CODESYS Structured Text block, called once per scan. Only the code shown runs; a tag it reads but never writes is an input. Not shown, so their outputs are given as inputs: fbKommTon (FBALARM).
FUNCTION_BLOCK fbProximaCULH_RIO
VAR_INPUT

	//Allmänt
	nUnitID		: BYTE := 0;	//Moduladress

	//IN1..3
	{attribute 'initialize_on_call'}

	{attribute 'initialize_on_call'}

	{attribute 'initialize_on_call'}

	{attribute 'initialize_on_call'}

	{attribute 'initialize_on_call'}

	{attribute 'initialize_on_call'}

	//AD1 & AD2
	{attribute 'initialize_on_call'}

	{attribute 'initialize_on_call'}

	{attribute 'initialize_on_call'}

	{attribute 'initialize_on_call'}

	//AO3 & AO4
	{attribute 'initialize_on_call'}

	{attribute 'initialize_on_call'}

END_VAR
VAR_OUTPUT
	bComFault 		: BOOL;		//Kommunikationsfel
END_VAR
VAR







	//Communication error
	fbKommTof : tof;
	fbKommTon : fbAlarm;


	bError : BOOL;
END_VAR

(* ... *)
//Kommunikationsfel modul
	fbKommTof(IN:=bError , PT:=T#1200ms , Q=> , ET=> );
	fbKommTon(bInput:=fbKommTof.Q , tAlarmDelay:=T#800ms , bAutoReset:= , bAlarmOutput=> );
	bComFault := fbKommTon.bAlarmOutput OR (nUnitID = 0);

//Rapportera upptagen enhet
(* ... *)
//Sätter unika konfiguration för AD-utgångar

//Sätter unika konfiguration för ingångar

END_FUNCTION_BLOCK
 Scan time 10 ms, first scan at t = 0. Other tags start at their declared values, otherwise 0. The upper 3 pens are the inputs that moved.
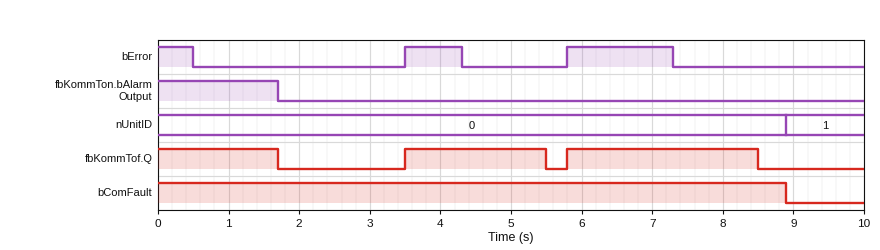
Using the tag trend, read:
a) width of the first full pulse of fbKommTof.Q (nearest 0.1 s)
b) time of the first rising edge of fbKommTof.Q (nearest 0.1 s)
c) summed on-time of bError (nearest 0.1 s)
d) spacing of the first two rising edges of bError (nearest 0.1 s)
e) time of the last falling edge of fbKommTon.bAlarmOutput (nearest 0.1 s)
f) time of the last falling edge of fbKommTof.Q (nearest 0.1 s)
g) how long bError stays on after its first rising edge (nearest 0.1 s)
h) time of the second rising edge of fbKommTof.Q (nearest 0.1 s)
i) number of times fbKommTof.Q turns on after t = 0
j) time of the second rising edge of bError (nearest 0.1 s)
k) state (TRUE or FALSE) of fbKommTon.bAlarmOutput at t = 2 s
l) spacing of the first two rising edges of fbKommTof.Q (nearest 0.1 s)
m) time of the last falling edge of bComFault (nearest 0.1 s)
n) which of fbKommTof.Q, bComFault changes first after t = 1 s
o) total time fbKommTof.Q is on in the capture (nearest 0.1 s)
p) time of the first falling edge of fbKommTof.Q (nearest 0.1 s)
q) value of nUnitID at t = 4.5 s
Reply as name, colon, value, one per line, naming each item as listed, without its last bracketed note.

width of the first full pulse of fbKommTof.Q: 2.0 s
time of the first rising edge of fbKommTof.Q: 3.5 s
summed on-time of bError: 2.8 s
spacing of the first two rising edges of bError: 2.3 s
time of the last falling edge of fbKommTon.bAlarmOutput: 1.7 s
time of the last falling edge of fbKommTof.Q: 8.5 s
how long bError stays on after its first rising edge: 0.8 s
time of the second rising edge of fbKommTof.Q: 5.8 s
number of times fbKommTof.Q turns on after t = 0: 2
time of the second rising edge of bError: 5.8 s
state (TRUE or FALSE) of fbKommTon.bAlarmOutput at t = 2 s: FALSE
spacing of the first two rising edges of fbKommTof.Q: 2.3 s
time of the last falling edge of bComFault: 8.9 s
which of fbKommTof.Q, bComFault changes first after t = 1 s: fbKommTof.Q
total time fbKommTof.Q is on in the capture: 6.4 s
time of the first falling edge of fbKommTof.Q: 1.7 s
value of nUnitID at t = 4.5 s: 0
